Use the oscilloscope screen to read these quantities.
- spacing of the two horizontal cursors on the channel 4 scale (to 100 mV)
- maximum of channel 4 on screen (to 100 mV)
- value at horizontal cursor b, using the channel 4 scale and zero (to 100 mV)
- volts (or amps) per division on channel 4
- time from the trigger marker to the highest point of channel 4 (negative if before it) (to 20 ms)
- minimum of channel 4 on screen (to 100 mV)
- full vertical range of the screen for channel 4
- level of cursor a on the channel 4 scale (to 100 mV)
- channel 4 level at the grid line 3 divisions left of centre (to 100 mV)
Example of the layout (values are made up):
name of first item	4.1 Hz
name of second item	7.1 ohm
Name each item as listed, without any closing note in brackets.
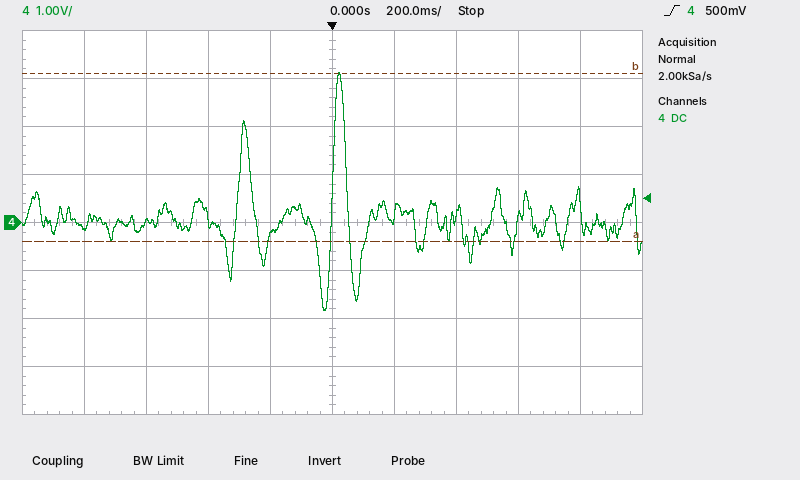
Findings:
spacing of the two horizontal cursors on the channel 4 scale	3.5 V
maximum of channel 4 on screen	3.1 V
value at horizontal cursor b, using the channel 4 scale and zero	3.1 V
volts (or amps) per division on channel 4	1 V
time from the trigger marker to the highest point of channel 4 (negative if before it)	+20 ms
minimum of channel 4 on screen	-1.8 V
full vertical range of the screen for channel 4	8 V
level of cursor a on the channel 4 scale	-400 mV
channel 4 level at the grid line 3 divisions left of centre	0.0 V
